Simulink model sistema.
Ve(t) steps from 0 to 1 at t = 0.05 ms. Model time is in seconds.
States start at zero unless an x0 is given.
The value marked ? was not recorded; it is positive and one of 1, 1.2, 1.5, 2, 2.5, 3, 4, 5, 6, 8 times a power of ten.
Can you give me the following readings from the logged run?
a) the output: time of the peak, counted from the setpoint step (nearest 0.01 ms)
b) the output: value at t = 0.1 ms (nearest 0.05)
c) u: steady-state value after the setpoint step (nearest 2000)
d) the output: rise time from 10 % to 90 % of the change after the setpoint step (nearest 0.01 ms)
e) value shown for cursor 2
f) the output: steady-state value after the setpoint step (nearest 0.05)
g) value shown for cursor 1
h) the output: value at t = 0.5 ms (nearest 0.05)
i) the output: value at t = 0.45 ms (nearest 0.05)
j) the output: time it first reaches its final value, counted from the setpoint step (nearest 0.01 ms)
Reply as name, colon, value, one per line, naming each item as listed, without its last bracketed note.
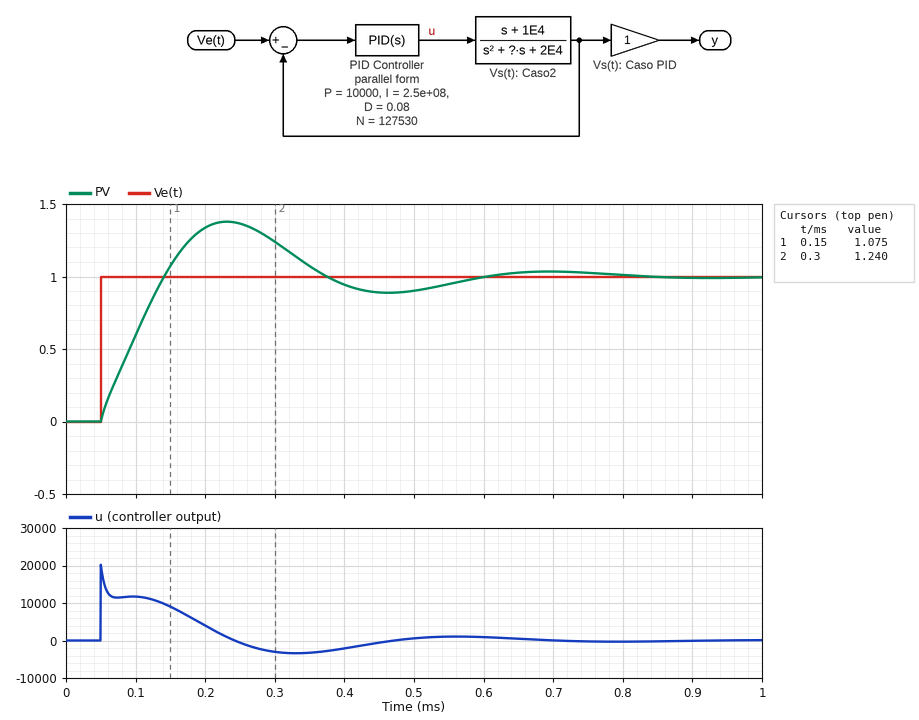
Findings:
the output: time of the peak, counted from the setpoint step: 0.18 ms
the output: value at t = 0.1 ms: 0.60
u: steady-state value after the setpoint step: 0
the output: rise time from 10 % to 90 % of the change after the setpoint step: 0.07 ms
value shown for cursor 2: 1.240
the output: steady-state value after the setpoint step: 1.00
value shown for cursor 1: 1.075
the output: value at t = 0.5 ms: 0.90
the output: value at t = 0.45 ms: 0.90
the output: time it first reaches its final value, counted from the setpoint step: 0.09 ms
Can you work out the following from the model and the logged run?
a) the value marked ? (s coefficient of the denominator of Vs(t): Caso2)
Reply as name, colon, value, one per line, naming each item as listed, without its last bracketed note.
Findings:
the value marked ? (s coefficient of the denominator of Vs(t): Caso2): 12000
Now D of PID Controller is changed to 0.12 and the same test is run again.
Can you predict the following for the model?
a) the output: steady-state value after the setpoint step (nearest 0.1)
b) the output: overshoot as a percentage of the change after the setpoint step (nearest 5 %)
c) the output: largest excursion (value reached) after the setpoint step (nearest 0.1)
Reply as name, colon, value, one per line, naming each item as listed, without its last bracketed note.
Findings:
the output: steady-state value after the setpoint step: 1.0
the output: overshoot as a percentage of the change after the setpoint step: 35 %
the output: largest excursion (value reached) after the setpoint step: 1.4
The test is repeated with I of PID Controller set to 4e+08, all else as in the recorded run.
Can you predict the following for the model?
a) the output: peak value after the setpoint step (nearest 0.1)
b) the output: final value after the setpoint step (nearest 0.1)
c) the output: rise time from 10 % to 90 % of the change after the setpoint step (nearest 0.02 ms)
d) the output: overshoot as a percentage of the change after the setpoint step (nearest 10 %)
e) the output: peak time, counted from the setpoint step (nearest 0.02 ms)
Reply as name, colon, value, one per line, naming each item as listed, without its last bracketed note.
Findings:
the output: peak value after the setpoint step: 1.4
the output: final value after the setpoint step: 1.0
the output: rise time from 10 % to 90 % of the change after the setpoint step: 0.06 ms
the output: overshoot as a percentage of the change after the setpoint step: 40 %
the output: peak time, counted from the setpoint step: 0.14 ms
